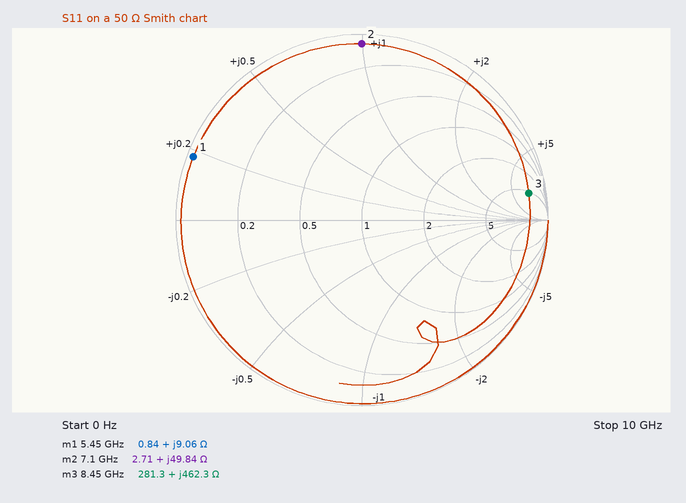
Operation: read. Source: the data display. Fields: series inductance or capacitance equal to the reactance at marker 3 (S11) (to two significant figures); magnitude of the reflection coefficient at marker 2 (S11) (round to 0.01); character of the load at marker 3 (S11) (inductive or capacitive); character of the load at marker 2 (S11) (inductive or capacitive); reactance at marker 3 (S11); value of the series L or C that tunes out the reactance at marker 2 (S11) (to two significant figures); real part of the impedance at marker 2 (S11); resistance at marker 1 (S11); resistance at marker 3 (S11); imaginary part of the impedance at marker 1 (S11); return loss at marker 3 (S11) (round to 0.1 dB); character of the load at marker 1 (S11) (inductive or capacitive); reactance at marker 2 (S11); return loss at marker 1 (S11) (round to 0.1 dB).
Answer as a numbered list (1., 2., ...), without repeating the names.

1. 8.7 nH
2. 0.95
3. inductive
4. inductive
5. +462.3 Ω
6. 450 fF
7. 2.71 Ω
8. 0.84 Ω
9. 281.3 Ω
10. +9.06 Ω
11. 0.8 dB
12. inductive
13. +49.84 Ω
14. 0.3 dB
